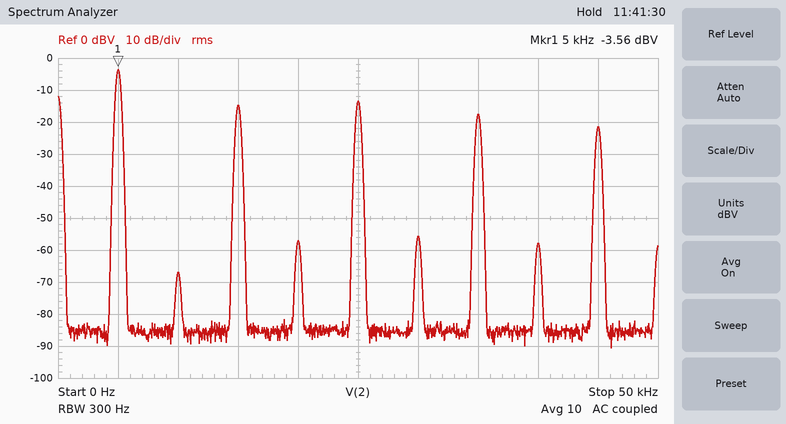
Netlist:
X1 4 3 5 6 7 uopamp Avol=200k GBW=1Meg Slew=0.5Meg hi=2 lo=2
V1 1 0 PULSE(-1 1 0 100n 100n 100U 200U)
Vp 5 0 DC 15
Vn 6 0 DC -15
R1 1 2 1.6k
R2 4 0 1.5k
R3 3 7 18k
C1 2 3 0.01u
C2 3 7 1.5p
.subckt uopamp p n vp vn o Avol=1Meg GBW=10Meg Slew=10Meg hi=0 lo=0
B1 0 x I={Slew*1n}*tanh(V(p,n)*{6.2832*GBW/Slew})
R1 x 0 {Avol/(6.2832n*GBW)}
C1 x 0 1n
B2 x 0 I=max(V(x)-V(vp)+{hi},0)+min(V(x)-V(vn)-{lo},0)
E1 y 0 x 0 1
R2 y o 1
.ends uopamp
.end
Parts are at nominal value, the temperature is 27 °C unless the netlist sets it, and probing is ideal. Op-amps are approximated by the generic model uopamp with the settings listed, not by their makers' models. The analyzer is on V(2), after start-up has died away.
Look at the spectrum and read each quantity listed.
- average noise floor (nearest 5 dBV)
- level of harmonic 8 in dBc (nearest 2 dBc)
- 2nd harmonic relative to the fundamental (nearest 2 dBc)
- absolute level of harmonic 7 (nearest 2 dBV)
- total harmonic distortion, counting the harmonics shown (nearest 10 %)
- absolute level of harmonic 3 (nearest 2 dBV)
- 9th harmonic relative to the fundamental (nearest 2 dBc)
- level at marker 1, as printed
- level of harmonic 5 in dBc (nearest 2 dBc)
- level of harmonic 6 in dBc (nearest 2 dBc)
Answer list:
-85 dBV
-54 dBc
-64 dBc
-18 dBV
50 %
-14 dBV
-18 dBc
-3.56 dBV
-10 dBc
-52 dBc
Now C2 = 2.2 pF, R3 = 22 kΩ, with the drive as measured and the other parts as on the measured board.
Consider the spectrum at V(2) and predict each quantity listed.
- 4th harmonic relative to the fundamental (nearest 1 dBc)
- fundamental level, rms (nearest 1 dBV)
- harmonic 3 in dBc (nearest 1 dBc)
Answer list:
-52 dBc
-4 dBV
-8 dBc
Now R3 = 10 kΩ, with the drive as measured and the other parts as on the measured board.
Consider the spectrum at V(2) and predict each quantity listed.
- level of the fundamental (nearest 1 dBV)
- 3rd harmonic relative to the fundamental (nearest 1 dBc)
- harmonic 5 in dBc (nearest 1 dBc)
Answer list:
-3 dBV
-20 dBc
-15 dBc
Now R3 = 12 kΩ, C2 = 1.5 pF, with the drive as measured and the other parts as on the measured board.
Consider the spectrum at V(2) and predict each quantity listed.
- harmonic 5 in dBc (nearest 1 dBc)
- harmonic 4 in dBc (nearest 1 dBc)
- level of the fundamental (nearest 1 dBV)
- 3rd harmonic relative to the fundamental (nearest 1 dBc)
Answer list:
-13 dBc
-58 dBc
-3 dBV
-17 dBc
